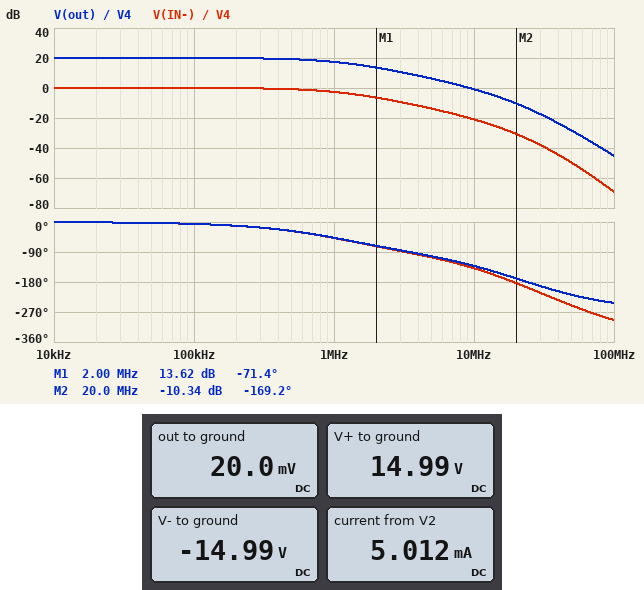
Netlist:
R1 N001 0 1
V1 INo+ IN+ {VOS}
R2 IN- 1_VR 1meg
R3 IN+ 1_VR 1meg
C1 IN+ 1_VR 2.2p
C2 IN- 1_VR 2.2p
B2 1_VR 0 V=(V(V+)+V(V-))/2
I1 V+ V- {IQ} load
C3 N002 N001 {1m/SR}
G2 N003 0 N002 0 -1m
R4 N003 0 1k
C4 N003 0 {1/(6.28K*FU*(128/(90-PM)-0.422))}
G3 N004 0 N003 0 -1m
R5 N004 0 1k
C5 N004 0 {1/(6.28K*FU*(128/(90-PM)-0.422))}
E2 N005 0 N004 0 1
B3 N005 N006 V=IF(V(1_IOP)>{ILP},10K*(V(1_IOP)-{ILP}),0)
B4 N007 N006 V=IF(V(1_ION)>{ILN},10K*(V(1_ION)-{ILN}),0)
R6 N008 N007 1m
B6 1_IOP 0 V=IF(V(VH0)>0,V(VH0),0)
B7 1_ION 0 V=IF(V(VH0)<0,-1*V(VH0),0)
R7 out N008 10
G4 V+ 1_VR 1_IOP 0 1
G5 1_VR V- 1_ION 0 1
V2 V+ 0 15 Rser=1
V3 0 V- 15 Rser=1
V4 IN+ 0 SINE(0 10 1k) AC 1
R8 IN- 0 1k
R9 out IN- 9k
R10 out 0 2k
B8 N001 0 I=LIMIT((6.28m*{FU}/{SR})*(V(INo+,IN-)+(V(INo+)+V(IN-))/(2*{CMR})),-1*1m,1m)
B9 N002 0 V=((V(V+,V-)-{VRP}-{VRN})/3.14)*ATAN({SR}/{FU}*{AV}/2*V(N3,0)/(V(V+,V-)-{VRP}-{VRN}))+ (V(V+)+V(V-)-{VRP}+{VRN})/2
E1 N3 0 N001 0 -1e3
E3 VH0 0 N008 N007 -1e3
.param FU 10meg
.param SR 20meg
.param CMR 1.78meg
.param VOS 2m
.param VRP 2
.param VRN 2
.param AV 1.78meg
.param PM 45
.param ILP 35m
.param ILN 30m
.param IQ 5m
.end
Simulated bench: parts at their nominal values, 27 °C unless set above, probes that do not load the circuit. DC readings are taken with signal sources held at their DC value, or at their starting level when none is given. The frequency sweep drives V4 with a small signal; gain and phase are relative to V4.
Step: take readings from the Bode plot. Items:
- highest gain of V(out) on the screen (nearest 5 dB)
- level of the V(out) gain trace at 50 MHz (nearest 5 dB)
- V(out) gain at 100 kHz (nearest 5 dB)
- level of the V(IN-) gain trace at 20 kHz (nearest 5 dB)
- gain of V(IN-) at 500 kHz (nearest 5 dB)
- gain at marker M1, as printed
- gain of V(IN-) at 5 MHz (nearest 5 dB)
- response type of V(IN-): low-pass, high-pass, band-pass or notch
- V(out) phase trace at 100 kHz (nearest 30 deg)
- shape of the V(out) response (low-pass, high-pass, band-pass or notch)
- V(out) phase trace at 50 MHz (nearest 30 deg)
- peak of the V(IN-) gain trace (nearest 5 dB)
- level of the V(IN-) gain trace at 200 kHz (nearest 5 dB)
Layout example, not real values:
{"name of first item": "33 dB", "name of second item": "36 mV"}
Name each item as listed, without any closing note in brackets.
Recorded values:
{"highest gain of V(out) on the screen": "20 dB", "level of the V(out) gain trace at 50 MHz": "-30 dB", "V(out) gain at 100 kHz": "20 dB", "level of the V(IN-) gain trace at 20 kHz": "0 dB", "gain of V(IN-) at 500 kHz": "0 dB", "gain at marker M1, as printed": "13.62 dB", "gain of V(IN-) at 5 MHz": "-15 dB", "response type of V(IN-): low-pass, high-pass, band-pass or notch": "low-pass", "V(out) phase trace at 100 kHz": "0 deg", "shape of the V(out) response": "low-pass", "V(out) phase trace at 50 MHz": "-210 deg", "peak of the V(IN-) gain trace": "0 dB", "level of the V(IN-) gain trace at 200 kHz": "0 dB"}
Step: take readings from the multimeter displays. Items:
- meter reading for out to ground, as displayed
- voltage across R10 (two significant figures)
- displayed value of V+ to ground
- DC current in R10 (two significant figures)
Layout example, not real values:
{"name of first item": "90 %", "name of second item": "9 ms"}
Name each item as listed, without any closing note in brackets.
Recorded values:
{"meter reading for out to ground, as displayed": "20.0 mV", "voltage across R10": "20 mV", "displayed value of V+ to ground": "14.99 V", "DC current in R10": "10 µA"}
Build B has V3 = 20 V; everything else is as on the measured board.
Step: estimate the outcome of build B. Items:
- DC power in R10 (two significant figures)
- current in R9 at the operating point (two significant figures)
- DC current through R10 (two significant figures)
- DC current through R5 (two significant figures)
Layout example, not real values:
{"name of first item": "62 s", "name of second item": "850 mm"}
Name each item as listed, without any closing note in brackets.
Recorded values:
{"DC power in R10": "900 nW", "current in R9 at the operating point": "4.5 µA", "DC current through R10": "21 µA", "DC current through R5": "43 µA"}
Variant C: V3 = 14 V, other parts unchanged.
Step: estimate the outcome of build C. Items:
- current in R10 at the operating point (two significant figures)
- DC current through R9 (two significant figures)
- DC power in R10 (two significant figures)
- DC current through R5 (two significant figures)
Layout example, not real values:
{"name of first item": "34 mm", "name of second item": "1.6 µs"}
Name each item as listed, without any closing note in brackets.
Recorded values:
{"current in R10 at the operating point": "7.8 µA", "DC current through R9": "1.5 µA", "DC power in R10": "120 nW", "DC current through R5": "16 µA"}
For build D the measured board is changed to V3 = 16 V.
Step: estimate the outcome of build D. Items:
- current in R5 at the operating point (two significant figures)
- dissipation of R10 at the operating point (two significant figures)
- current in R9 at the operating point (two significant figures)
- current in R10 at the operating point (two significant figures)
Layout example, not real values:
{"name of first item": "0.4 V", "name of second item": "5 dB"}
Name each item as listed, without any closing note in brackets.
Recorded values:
{"current in R5 at the operating point": "25 µA", "dissipation of R10 at the operating point": "300 nW", "current in R9 at the operating point": "2.5 µA", "current in R10 at the operating point": "12 µA"}
